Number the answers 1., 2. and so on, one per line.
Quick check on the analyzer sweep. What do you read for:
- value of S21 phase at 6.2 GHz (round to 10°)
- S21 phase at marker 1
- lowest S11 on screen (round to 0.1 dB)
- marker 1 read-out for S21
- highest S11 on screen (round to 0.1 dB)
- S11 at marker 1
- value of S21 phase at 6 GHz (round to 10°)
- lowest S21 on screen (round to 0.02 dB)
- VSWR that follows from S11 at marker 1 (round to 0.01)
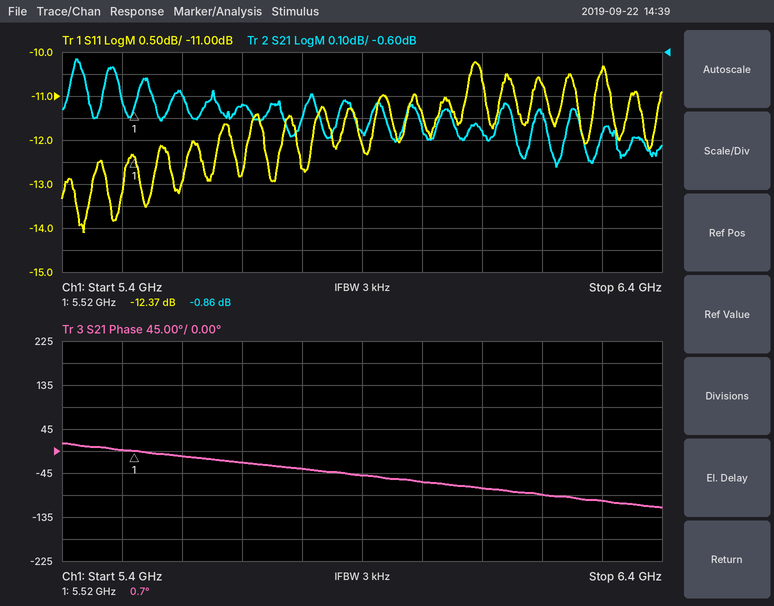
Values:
1. -90°
2. 0.7°
3. -14.1 dB
4. -0.86 dB
5. -10.2 dB
6. -12.37 dB
7. -60°
8. -1.12 dB
9. 1.63
